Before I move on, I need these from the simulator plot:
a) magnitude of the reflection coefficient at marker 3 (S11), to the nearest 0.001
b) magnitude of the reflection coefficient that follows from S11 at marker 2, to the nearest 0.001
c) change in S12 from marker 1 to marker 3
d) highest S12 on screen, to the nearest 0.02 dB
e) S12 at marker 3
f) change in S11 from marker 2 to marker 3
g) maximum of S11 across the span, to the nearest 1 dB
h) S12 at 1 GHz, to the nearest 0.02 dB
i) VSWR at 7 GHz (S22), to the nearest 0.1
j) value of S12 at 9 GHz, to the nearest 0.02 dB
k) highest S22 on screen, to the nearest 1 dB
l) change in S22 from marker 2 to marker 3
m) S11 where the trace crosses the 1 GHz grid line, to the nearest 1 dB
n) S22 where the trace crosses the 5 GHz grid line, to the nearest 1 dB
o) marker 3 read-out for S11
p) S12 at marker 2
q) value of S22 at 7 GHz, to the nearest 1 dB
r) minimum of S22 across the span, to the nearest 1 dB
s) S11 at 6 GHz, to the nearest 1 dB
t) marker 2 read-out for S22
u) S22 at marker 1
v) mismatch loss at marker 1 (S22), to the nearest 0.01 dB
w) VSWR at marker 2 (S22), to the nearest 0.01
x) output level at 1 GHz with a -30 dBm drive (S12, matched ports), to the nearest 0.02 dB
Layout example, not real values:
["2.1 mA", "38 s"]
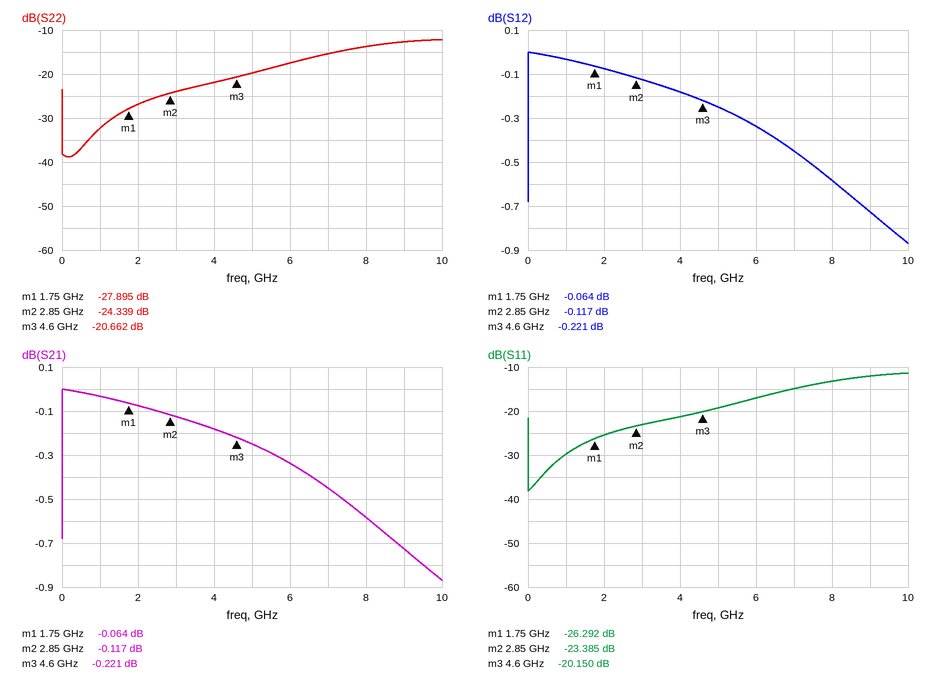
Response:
["0.098", "0.068", "-0.157 dB", "0.00 dB", "-0.221 dB", "3.235 dB", "-11 dB", "-0.04 dB", "1.4", "-0.72 dB", "-12 dB", "3.677 dB", "-30 dB", "-20 dB", "-20.150 dB", "-0.117 dB", "-15 dB", "-39 dB", "-17 dB", "-24.339 dB", "-27.895 dB", "0.01 dB", "1.13", "-30.04 dBm"]
